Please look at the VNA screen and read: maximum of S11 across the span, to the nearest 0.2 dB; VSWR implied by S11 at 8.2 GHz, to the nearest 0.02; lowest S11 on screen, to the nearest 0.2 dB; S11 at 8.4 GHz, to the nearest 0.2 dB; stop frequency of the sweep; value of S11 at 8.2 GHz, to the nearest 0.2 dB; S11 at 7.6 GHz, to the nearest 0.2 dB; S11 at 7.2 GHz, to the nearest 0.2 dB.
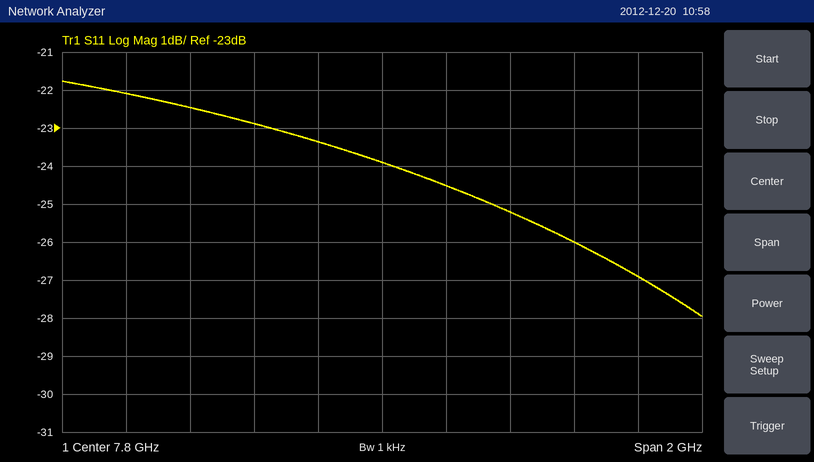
-21.8 dB
1.12
-28.0 dB
-26.0 dB
8.8 GHz
-25.2 dB
-23.4 dB
-22.4 dB
